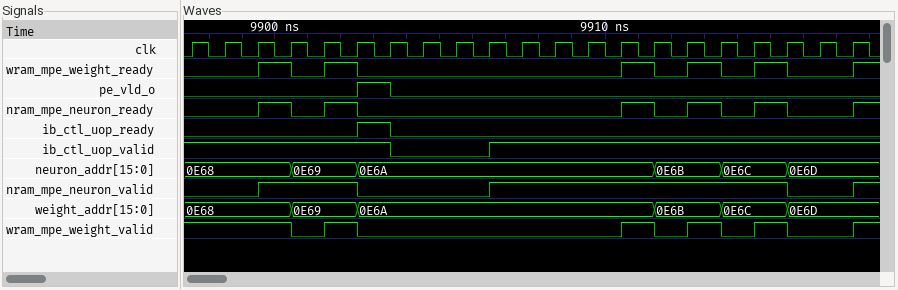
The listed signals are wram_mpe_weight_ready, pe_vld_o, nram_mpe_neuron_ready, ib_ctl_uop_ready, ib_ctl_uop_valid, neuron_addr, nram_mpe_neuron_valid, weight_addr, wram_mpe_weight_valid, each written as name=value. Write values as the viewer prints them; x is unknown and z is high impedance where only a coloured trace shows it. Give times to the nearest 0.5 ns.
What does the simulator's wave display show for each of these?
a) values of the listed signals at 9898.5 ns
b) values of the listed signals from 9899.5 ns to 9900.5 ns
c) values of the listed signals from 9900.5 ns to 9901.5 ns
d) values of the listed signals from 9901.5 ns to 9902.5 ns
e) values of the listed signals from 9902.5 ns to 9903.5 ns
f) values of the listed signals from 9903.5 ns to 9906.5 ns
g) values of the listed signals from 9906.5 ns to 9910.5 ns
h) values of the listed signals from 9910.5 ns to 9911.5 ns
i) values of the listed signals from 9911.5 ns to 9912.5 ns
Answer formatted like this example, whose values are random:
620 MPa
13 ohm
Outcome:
wram_mpe_weight_ready=0, pe_vld_o=0, nram_mpe_neuron_ready=0, ib_ctl_uop_ready=0, ib_ctl_uop_valid=1, neuron_addr=0E68, nram_mpe_neuron_valid=0, weight_addr=0E68, wram_mpe_weight_valid=1
wram_mpe_weight_ready=1, pe_vld_o=0, nram_mpe_neuron_ready=1, ib_ctl_uop_ready=0, ib_ctl_uop_valid=1, neuron_addr=0E68, nram_mpe_neuron_valid=1, weight_addr=0E68, wram_mpe_weight_valid=1
wram_mpe_weight_ready=0, pe_vld_o=0, nram_mpe_neuron_ready=0, ib_ctl_uop_ready=0, ib_ctl_uop_valid=1, neuron_addr=0E69, nram_mpe_neuron_valid=1, weight_addr=0E69, wram_mpe_weight_valid=0
wram_mpe_weight_ready=1, pe_vld_o=0, nram_mpe_neuron_ready=1, ib_ctl_uop_ready=0, ib_ctl_uop_valid=1, neuron_addr=0E69, nram_mpe_neuron_valid=1, weight_addr=0E69, wram_mpe_weight_valid=1
wram_mpe_weight_ready=0, pe_vld_o=1, nram_mpe_neuron_ready=0, ib_ctl_uop_ready=1, ib_ctl_uop_valid=1, neuron_addr=0E6A, nram_mpe_neuron_valid=0, weight_addr=0E6A, wram_mpe_weight_valid=0
wram_mpe_weight_ready=0, pe_vld_o=0, nram_mpe_neuron_ready=0, ib_ctl_uop_ready=0, ib_ctl_uop_valid=0, neuron_addr=0E6A, nram_mpe_neuron_valid=0, weight_addr=0E6A, wram_mpe_weight_valid=0
wram_mpe_weight_ready=0, pe_vld_o=0, nram_mpe_neuron_ready=0, ib_ctl_uop_ready=0, ib_ctl_uop_valid=1, neuron_addr=0E6A, nram_mpe_neuron_valid=1, weight_addr=0E6A, wram_mpe_weight_valid=0
wram_mpe_weight_ready=1, pe_vld_o=0, nram_mpe_neuron_ready=1, ib_ctl_uop_ready=0, ib_ctl_uop_valid=1, neuron_addr=0E6A, nram_mpe_neuron_valid=1, weight_addr=0E6A, wram_mpe_weight_valid=1
wram_mpe_weight_ready=0, pe_vld_o=0, nram_mpe_neuron_ready=0, ib_ctl_uop_ready=0, ib_ctl_uop_valid=1, neuron_addr=0E6B, nram_mpe_neuron_valid=1, weight_addr=0E6B, wram_mpe_weight_valid=0
